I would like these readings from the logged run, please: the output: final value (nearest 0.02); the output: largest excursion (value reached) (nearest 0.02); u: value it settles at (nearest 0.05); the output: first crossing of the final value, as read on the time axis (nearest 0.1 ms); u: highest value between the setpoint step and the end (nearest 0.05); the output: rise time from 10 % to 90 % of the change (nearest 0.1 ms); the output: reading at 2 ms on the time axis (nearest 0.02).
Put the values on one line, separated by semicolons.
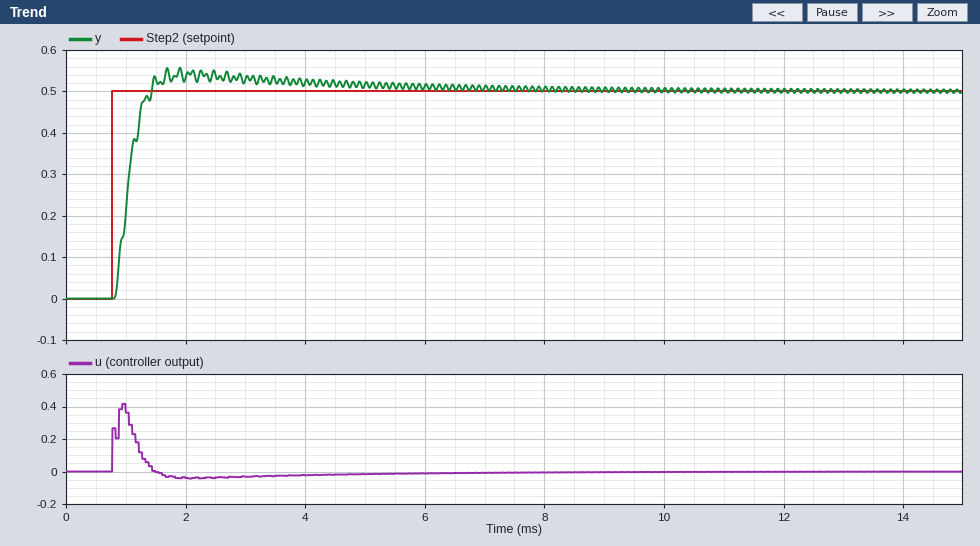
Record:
0.50; 0.56; 0.00; 1.4 ms; 0.40; 0.4 ms; 0.54
